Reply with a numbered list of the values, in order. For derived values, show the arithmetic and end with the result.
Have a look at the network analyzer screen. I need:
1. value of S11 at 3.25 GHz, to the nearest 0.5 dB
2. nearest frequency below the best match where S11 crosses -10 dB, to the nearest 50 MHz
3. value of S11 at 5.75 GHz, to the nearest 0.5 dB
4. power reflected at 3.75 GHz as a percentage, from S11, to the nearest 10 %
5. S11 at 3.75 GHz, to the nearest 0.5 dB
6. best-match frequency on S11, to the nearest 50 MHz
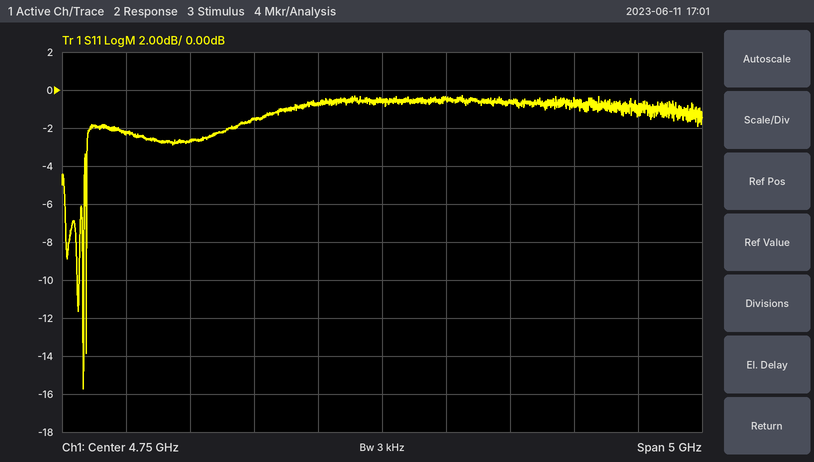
1. -2.5 dB
2. 2.40 GHz
3. -0.5 dB
4. 10^(-1.5/10) ≈ 70.8 %, so 70 % to the nearest 10 %
5. -1.5 dB
6. 2.40 GHz
